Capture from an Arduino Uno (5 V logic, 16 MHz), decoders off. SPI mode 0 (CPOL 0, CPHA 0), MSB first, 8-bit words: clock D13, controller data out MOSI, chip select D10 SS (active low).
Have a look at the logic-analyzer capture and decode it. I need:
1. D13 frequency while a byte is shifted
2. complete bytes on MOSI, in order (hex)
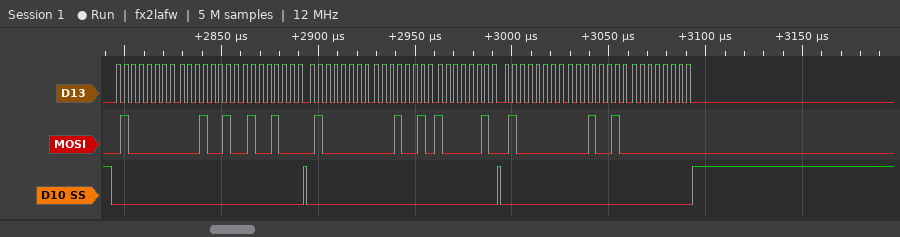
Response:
250 kHz
40 12 48 40 12 82 40 12 00
